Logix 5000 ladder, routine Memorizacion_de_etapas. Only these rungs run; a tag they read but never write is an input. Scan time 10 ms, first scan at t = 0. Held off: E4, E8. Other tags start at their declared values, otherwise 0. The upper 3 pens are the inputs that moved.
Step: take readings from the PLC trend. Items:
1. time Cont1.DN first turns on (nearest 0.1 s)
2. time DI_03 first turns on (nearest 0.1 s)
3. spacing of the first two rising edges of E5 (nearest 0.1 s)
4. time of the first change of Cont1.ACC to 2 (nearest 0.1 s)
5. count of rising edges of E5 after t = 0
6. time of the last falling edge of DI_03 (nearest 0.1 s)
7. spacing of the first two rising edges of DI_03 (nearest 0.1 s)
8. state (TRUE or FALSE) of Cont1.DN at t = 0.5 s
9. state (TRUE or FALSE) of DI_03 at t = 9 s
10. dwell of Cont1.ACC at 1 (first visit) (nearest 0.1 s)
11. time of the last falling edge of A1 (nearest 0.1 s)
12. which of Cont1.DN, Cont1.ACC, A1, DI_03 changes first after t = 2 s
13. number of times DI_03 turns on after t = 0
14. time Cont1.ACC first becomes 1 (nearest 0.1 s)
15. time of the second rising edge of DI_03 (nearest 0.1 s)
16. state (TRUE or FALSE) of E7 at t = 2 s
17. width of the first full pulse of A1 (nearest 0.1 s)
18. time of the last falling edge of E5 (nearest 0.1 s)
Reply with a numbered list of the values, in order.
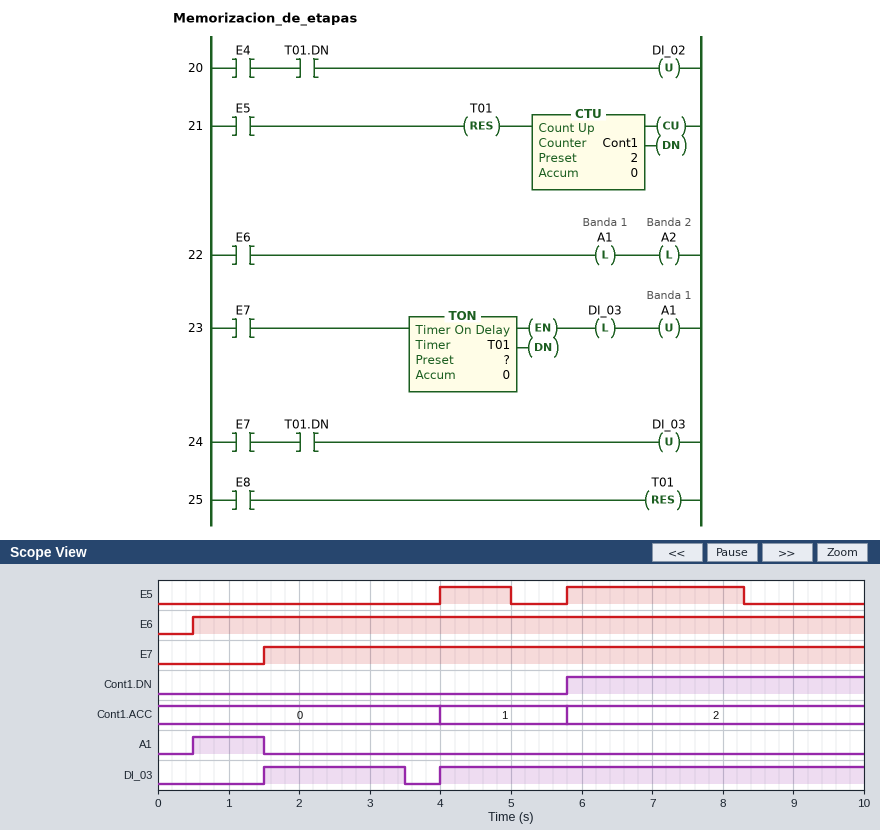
1. 5.8 s
2. 1.5 s
3. 1.8 s
4. 5.8 s
5. 2
6. 3.5 s
7. 2.5 s
8. FALSE
9. TRUE
10. 1.8 s
11. 1.5 s
12. DI_03
13. 2
14. 4.0 s
15. 4.0 s
16. TRUE
17. 1.0 s
18. 8.3 s
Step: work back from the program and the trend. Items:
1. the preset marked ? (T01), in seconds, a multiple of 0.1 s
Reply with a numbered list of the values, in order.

1. 2.0 s
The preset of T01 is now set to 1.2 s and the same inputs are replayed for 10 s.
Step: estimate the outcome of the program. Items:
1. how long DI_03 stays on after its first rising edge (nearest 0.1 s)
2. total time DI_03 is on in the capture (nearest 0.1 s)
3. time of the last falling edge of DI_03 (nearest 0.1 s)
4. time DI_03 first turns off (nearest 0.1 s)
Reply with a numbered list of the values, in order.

1. 1.2 s
2. 6.7 s
3. 9.5 s
4. 2.7 s
